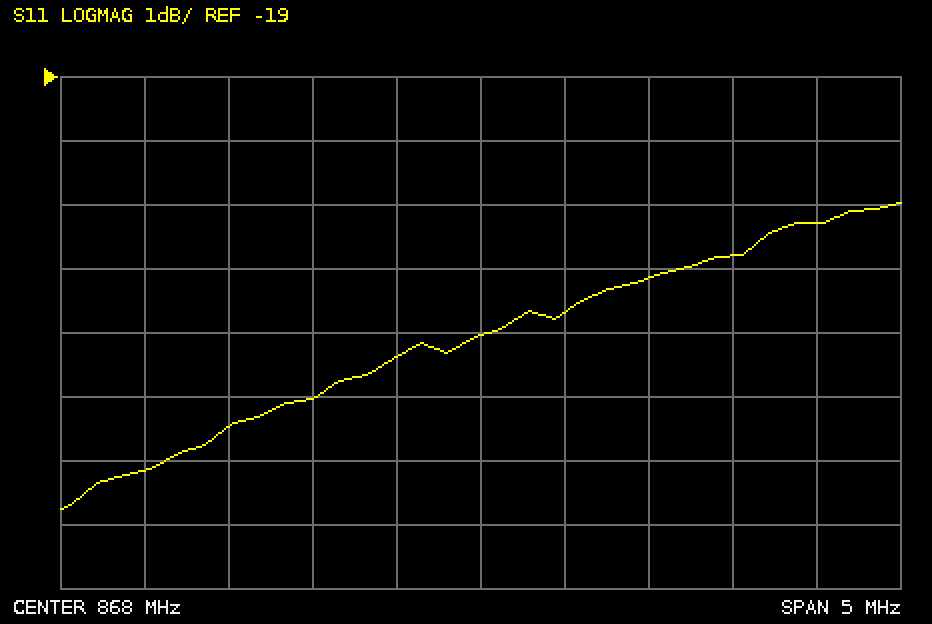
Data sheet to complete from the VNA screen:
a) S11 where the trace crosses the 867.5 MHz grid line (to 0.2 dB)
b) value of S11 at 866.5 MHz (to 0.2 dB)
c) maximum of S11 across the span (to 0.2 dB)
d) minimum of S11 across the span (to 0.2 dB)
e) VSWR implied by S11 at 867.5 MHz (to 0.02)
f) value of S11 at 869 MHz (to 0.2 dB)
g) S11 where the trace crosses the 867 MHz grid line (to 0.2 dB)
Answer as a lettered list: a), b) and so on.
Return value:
a) -23.4 dB
b) -24.4 dB
c) -21.0 dB
d) -25.8 dB
e) 1.14
f) -22.2 dB
g) -24.0 dB
